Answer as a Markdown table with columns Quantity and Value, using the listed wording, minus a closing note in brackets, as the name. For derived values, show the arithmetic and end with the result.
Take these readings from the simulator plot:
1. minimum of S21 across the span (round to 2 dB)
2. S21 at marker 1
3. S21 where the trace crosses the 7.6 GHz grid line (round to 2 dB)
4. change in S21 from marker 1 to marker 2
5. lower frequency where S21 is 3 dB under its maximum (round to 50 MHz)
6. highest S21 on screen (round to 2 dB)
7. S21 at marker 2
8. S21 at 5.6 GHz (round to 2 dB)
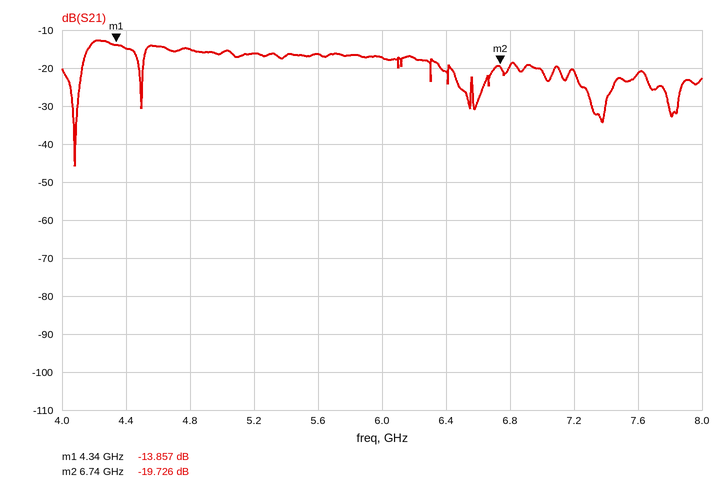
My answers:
| Quantity | Value |
|---|---|
| minimum of S21 across the span | -46 dB |
| S21 at marker 1 | -13.857 dB |
| S21 where the trace crosses the 7.6 GHz grid line | -22 dB |
| change in S21 from marker 1 to marker 2 | -19.726 − (-13.857) = -5.869 dB |
| lower frequency where S21 is 3 dB under its maximum | 4.15 GHz |
| highest S21 on screen | -12 dB |
| S21 at marker 2 | -19.726 dB |
| S21 at 5.6 GHz | -16 dB |
